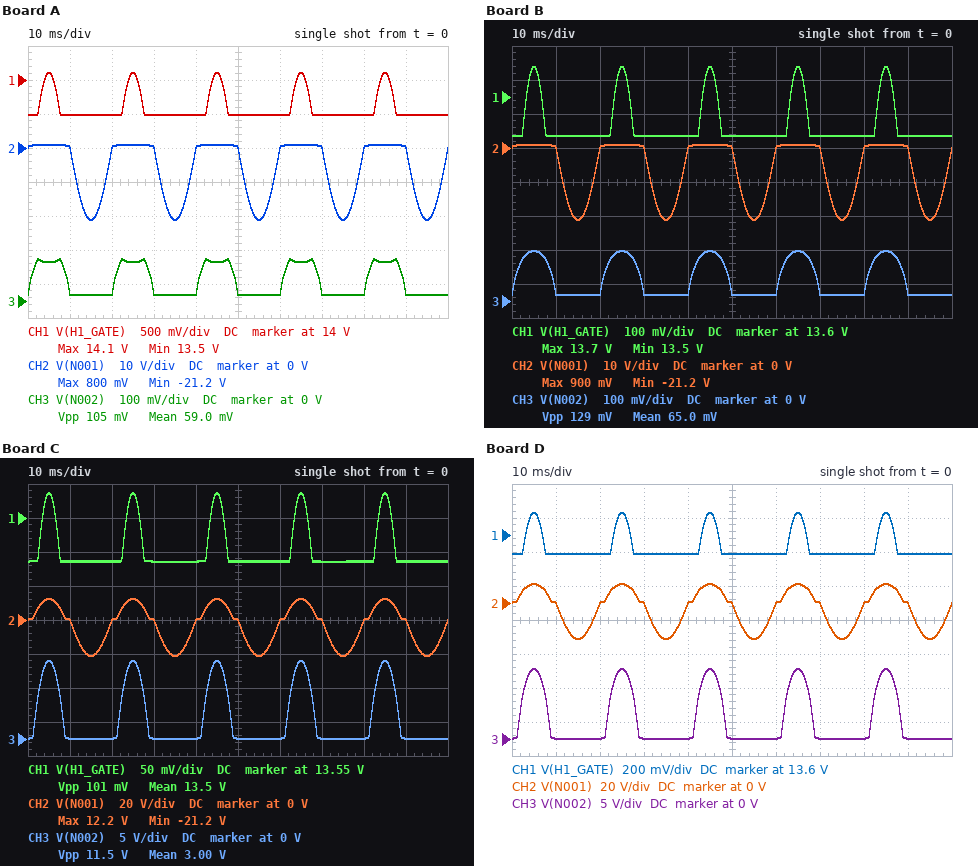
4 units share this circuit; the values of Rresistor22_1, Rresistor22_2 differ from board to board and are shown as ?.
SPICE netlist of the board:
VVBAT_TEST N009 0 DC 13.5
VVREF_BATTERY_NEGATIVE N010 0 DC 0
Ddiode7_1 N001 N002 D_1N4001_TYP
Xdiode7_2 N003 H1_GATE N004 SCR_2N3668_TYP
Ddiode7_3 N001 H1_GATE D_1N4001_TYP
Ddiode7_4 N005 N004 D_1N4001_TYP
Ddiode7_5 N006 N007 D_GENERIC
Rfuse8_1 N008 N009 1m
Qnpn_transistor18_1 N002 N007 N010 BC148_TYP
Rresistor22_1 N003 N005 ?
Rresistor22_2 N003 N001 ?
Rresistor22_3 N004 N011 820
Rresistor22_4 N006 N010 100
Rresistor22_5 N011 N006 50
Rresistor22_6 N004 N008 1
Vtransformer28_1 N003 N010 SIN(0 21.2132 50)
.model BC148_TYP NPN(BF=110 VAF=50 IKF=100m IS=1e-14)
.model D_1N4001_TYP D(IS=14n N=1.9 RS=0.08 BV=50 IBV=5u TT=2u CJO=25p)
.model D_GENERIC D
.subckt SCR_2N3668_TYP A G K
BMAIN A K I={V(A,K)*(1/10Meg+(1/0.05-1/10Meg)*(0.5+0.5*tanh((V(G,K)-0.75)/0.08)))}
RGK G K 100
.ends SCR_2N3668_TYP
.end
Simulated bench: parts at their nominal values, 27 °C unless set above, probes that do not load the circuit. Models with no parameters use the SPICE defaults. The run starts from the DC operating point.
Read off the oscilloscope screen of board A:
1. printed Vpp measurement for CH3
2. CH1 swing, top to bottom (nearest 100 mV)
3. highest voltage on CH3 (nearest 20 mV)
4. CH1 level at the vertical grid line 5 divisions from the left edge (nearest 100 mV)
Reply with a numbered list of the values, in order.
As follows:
1. 105 mV
2. 600 mV
3. 120 mV
4. 13.5 V
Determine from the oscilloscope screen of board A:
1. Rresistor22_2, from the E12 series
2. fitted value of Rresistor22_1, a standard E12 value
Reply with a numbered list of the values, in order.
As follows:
1. 820 Ω
2. 10 Ω
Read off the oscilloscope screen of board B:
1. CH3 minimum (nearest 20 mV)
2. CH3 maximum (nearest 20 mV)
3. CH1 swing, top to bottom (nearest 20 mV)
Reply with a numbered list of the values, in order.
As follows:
1. 20 mV
2. 140 mV
3. 200 mV
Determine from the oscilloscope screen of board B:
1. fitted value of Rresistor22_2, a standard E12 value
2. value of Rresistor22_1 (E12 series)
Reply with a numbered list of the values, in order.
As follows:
1. 820 Ω
2. 33 Ω
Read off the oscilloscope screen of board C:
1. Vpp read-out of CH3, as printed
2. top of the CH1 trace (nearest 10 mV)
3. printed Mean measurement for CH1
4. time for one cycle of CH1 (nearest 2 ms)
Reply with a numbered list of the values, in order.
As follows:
1. 11.5 V
2. 13.59 V
3. 13.5 V
4. 20 ms
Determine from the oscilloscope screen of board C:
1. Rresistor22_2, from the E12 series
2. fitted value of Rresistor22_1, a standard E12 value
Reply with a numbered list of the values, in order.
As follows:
1. 270 Ω
2. 68 Ω
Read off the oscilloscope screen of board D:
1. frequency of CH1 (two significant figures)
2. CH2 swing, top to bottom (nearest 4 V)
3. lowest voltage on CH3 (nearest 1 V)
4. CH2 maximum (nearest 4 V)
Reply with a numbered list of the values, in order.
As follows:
1. 50 Hz
2. 32 V
3. 0 V
4. 12 V
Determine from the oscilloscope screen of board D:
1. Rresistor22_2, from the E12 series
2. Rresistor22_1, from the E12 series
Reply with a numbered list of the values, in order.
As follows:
1. 270 Ω
2. 27 Ω
